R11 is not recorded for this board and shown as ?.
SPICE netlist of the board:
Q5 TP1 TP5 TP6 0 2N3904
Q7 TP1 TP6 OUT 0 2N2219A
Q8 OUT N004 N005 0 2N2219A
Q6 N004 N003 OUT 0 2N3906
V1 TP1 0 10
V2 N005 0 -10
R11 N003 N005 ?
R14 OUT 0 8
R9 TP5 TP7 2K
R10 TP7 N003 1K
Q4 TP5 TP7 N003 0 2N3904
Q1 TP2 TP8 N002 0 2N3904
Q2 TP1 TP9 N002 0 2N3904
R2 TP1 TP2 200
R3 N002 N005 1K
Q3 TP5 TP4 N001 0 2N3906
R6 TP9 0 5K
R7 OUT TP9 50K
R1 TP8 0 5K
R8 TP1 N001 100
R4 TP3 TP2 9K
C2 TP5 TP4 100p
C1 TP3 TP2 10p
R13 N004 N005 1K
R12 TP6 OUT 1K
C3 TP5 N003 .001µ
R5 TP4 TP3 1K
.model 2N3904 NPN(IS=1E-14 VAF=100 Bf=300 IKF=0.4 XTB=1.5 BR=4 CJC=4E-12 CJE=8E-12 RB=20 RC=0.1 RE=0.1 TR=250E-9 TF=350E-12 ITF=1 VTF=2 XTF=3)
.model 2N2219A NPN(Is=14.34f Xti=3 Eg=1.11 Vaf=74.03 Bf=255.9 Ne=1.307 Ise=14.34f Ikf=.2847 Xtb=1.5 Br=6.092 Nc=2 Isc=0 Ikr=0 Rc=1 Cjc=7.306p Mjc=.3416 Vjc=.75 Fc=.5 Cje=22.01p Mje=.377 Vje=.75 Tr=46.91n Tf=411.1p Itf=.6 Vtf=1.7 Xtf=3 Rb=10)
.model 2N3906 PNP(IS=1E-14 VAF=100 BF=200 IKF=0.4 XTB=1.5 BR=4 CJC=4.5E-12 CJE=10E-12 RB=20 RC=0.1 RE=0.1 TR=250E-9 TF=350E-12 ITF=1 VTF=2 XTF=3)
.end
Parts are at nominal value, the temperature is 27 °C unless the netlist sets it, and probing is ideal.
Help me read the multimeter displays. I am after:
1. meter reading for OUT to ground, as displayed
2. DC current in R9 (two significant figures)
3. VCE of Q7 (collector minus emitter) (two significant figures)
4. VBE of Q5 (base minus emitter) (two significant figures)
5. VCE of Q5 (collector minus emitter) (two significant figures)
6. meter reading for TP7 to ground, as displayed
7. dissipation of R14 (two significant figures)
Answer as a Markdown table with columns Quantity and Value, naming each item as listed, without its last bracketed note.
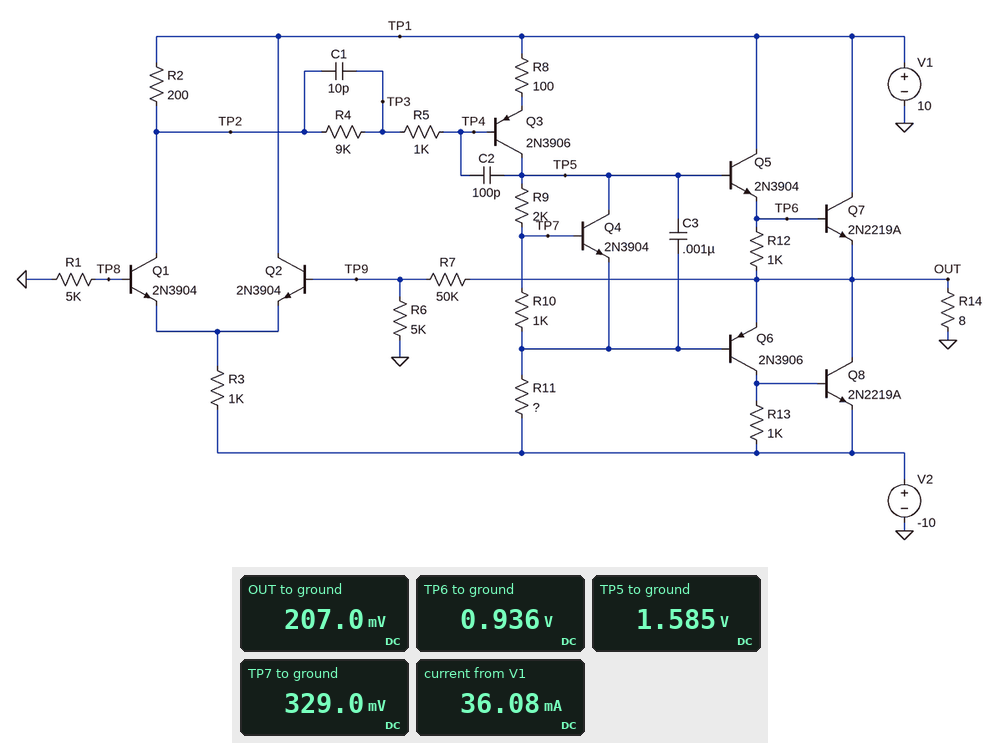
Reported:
| Quantity | Value |
|---|---|
| meter reading for OUT to ground, as displayed | 207.0 mV |
| DC current in R9 | 630 µA |
| VCE of Q7 (collector minus emitter) | 9.8 V |
| VBE of Q5 (base minus emitter) | 650 mV |
| VCE of Q5 (collector minus emitter) | 9.1 V |
| meter reading for TP7 to ground, as displayed | 329.0 mV |
| dissipation of R14 | 5.4 mW |
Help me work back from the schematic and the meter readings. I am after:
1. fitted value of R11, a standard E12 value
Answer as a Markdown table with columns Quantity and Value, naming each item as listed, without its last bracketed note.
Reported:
| Quantity | Value |
|---|---|
| fitted value of R11, a standard E12 value | 10 kΩ |
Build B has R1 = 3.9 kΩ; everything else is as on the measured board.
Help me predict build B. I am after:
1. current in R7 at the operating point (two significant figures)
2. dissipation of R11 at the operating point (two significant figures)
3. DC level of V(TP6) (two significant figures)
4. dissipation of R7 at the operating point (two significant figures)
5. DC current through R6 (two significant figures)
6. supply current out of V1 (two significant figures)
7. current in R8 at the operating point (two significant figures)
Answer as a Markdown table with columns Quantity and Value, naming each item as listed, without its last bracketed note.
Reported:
| Quantity | Value |
|---|---|
| current in R7 at the operating point | 7.9 µA |
| dissipation of R11 at the operating point | 9.7 mW |
| DC level of V(TP6) | 1.1 V |
| dissipation of R7 at the operating point | 3.1 µW |
| DC current through R6 | 8.2 µA |
| supply current out of V1 | 54 mA |
| current in R8 at the operating point | 990 µA |
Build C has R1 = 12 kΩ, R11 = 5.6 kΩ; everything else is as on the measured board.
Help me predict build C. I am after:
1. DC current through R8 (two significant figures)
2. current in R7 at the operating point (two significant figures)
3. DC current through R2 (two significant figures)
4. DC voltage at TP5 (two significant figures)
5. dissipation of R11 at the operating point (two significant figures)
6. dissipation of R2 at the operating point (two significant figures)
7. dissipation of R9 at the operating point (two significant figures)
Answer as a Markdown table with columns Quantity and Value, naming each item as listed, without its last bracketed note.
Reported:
| Quantity | Value |
|---|---|
| DC current through R8 | 1.5 mA |
| current in R7 at the operating point | 18 µA |
| DC current through R2 | 4.4 mA |
| DC voltage at TP5 | 240 mV |
| dissipation of R11 at the operating point | 12 mW |
| dissipation of R2 at the operating point | 3.9 mW |
| dissipation of R9 at the operating point | 850 µW |
